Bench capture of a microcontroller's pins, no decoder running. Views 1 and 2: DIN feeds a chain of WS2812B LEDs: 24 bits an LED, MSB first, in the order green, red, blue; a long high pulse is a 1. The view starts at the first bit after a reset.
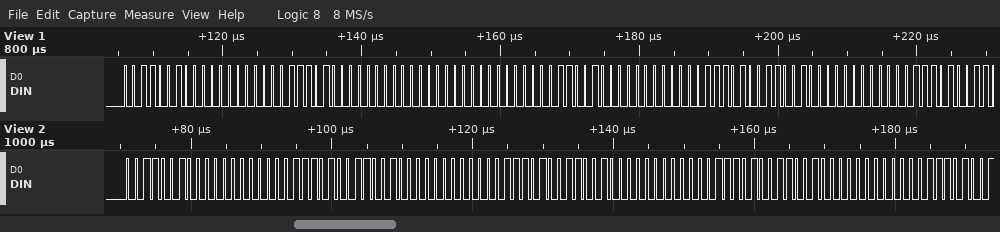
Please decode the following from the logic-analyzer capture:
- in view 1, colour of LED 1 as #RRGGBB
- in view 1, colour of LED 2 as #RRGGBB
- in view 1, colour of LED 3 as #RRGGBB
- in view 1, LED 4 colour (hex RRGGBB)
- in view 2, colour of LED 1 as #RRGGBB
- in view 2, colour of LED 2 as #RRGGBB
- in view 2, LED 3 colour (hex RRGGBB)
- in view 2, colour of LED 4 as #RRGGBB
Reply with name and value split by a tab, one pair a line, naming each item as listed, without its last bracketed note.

in view 1, colour of LED 1 as #RRGGBB	#00321D
in view 1, colour of LED 2 as #RRGGBB	#000000
in view 1, colour of LED 3 as #RRGGBB	#00321D
in view 1, LED 4 colour	#00321D
in view 2, colour of LED 1 as #RRGGBB	#00321D
in view 2, colour of LED 2 as #RRGGBB	#00321D
in view 2, LED 3 colour	#00321D
in view 2, colour of LED 4 as #RRGGBB	#00321D
